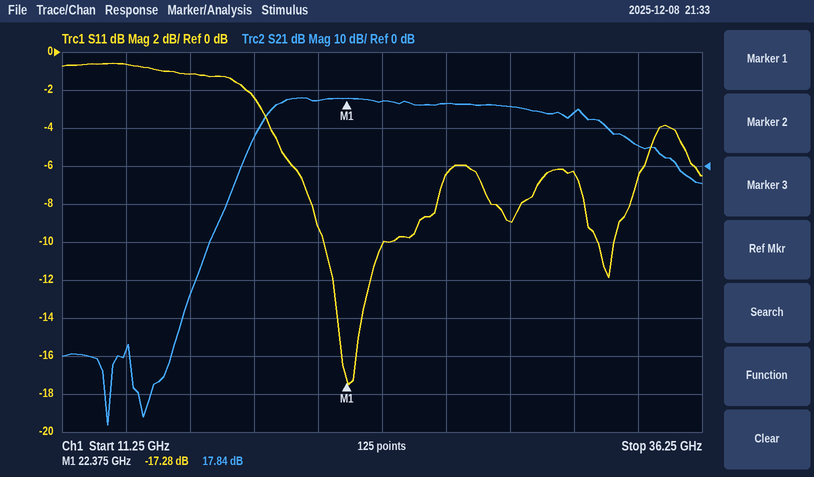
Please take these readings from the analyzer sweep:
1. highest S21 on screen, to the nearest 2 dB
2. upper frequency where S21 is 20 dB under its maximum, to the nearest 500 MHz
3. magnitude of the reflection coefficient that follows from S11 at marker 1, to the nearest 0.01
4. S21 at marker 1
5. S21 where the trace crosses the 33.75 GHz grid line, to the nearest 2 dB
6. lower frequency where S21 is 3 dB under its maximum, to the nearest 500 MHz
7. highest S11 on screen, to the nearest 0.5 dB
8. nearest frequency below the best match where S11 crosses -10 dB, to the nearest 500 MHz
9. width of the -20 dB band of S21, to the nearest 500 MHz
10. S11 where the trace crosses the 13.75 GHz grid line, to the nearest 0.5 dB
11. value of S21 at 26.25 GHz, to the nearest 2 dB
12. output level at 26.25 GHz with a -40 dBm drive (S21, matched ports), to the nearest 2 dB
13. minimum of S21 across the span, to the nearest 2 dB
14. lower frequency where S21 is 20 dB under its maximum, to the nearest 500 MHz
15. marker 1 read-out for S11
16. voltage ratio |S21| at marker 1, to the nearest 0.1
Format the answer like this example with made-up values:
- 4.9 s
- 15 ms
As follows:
- 18 dB
- 35.5 GHz
- 0.14
- 17.84 dB
- 6 dB
- 19.5 GHz
- -0.5 dB
- 21.5 GHz
- 17.5 GHz
- -0.5 dB
- 16 dB
- -24 dBm
- -68 dB
- 18.0 GHz
- -17.28 dB
- 7.8
